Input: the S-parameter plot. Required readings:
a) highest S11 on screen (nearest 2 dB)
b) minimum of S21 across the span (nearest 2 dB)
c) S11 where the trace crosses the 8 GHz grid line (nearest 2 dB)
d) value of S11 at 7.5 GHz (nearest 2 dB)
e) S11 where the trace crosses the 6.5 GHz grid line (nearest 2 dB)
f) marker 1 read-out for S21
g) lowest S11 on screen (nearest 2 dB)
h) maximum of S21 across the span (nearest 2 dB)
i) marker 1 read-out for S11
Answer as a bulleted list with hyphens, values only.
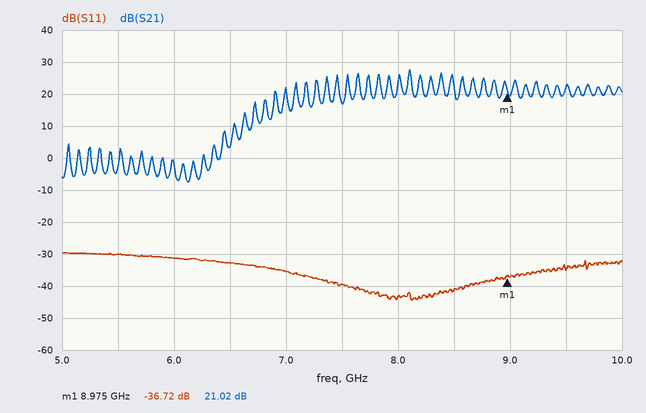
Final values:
- -30 dB
- -8 dB
- -44 dB
- -40 dB
- -32 dB
- 21.02 dB
- -44 dB
- 28 dB
- -36.72 dB
